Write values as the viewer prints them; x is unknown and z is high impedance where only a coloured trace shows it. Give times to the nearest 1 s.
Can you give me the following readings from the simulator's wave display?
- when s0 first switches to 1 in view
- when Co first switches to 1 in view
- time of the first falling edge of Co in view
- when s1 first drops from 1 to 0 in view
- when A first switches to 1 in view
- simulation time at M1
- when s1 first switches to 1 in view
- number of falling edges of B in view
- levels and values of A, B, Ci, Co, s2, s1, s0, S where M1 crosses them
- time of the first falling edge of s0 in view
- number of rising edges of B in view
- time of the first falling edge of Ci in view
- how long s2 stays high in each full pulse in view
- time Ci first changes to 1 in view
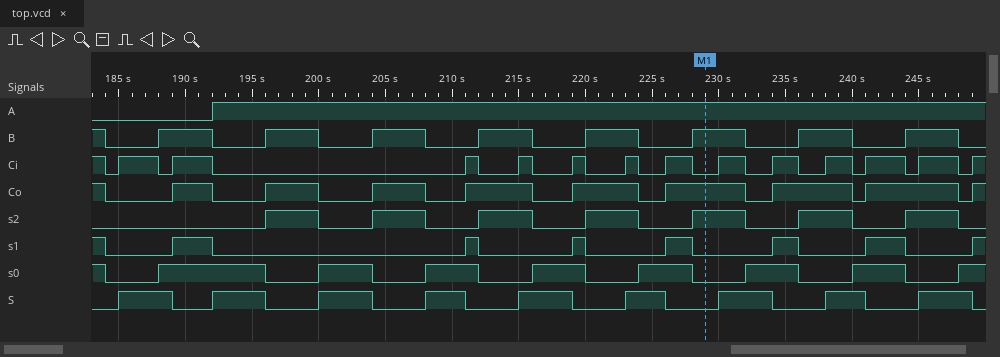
188 s
189 s
184 s
184 s
192 s
229 s
189 s
9
A=1, B=1, Ci=0, Co=1, s2=1, s1=0, s0=0, S=0
184 s
8
184 s
4 s, 4 s, 4 s, 4 s, 4 s, 4 s, 4 s
185 s
